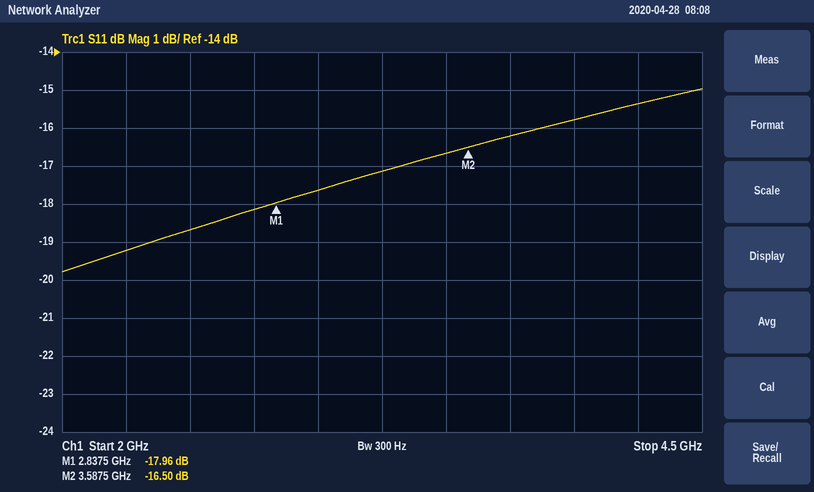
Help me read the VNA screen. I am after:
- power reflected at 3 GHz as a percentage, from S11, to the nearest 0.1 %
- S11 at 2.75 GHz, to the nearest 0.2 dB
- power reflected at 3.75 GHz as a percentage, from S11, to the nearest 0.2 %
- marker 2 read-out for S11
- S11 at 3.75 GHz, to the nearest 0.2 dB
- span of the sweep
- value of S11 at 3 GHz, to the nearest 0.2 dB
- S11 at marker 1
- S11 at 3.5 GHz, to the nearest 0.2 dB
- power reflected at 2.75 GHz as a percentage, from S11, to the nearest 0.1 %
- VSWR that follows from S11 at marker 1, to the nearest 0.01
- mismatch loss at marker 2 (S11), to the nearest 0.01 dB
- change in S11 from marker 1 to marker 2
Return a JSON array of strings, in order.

["1.7 %", "-18.2 dB", "2.4 %", "-16.50 dB", "-16.2 dB", "2.5 GHz", "-17.6 dB", "-17.96 dB", "-16.6 dB", "1.5 %", "1.29", "0.10 dB", "1.46 dB"]
